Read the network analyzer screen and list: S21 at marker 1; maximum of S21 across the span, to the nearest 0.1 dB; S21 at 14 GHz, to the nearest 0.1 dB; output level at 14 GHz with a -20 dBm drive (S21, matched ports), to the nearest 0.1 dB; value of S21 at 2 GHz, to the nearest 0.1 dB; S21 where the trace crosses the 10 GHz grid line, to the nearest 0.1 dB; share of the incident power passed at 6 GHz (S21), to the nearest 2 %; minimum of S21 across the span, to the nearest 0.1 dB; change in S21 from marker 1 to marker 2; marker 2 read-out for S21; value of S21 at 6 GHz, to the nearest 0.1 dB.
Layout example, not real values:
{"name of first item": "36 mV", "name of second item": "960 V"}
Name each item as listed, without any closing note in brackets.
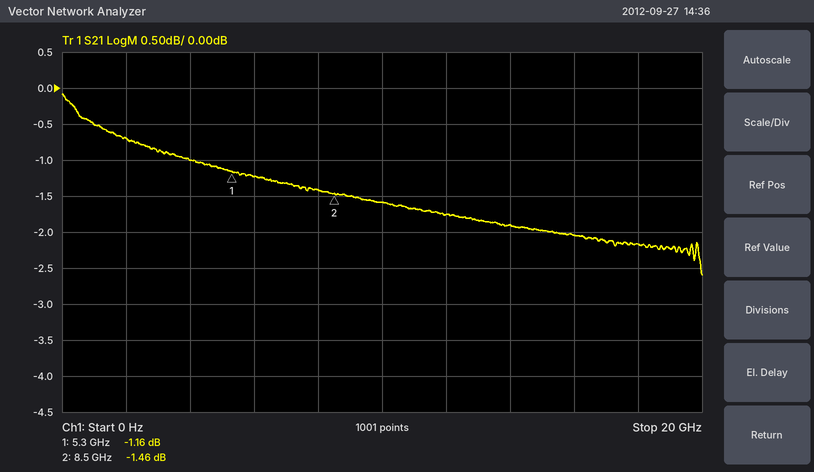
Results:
{"S21 at marker 1": "-1.16 dB", "maximum of S21 across the span, to the nearest 0.1 dB": "-0.1 dB", "S21 at 14 GHz, to the nearest 0.1 dB": "-1.9 dB", "output level at 14 GHz with a -20 dBm drive (S21, matched ports), to the nearest 0.1 dB": "-21.9 dBm", "value of S21 at 2 GHz, to the nearest 0.1 dB": "-0.7 dB", "S21 where the trace crosses the 10 GHz grid line, to the nearest 0.1 dB": "-1.6 dB", "share of the incident power passed at 6 GHz (S21), to the nearest 2 %": "76 %", "minimum of S21 across the span, to the nearest 0.1 dB": "-2.6 dB", "change in S21 from marker 1 to marker 2": "-0.30 dB", "marker 2 read-out for S21": "-1.46 dB", "value of S21 at 6 GHz, to the nearest 0.1 dB": "-1.2 dB"}
